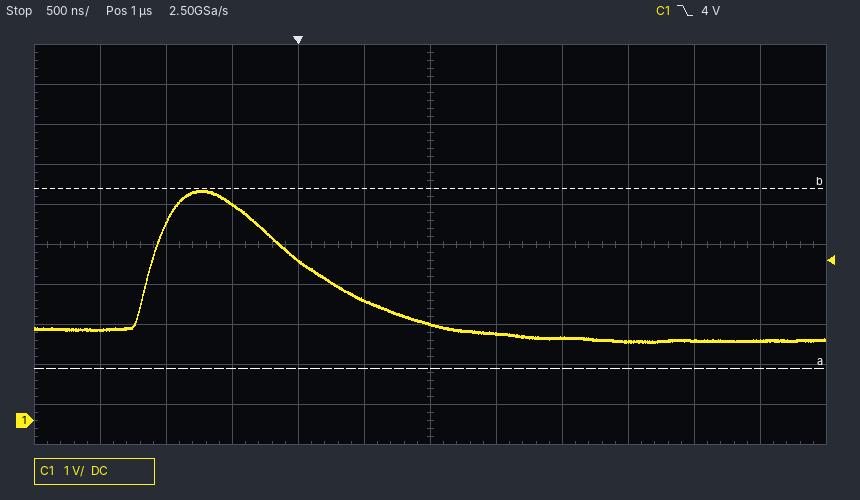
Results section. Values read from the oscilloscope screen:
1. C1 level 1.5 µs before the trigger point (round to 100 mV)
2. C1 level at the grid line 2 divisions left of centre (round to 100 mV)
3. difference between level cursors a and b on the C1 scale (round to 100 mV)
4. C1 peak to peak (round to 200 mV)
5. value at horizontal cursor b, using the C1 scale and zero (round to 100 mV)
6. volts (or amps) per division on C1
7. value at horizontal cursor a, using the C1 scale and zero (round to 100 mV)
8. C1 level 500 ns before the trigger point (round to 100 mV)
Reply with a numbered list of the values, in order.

1. 2.3 V
2. 4.0 V
3. 4.5 V
4. 3.8 V
5. 5.8 V
6. 1 V
7. 1.3 V
8. 5.4 V
